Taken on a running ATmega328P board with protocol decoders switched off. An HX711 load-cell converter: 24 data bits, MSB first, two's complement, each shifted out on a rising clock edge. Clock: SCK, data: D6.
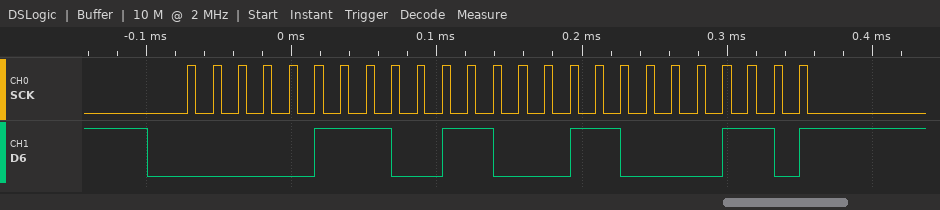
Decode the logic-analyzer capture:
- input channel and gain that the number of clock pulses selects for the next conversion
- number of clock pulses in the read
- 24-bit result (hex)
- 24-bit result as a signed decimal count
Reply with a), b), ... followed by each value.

a) channel A, gain 128
b) 25
c) 0x073186
d) 471430
